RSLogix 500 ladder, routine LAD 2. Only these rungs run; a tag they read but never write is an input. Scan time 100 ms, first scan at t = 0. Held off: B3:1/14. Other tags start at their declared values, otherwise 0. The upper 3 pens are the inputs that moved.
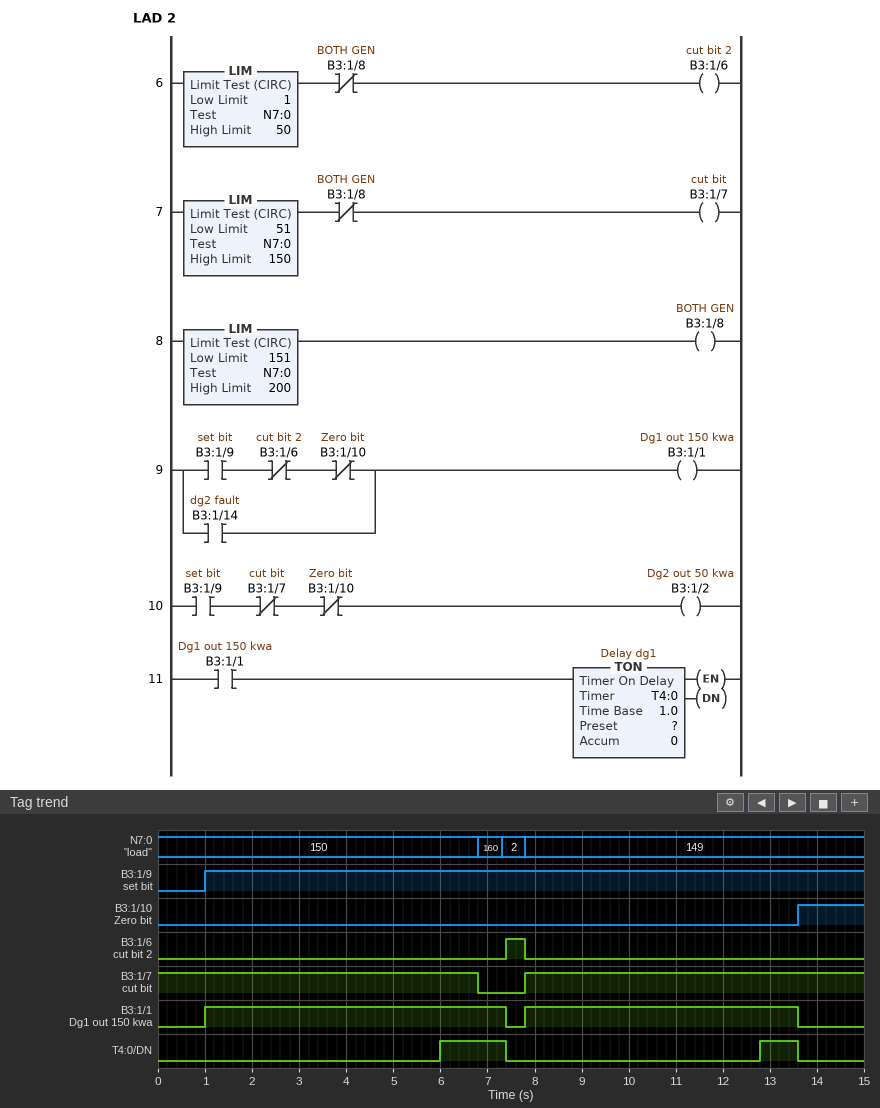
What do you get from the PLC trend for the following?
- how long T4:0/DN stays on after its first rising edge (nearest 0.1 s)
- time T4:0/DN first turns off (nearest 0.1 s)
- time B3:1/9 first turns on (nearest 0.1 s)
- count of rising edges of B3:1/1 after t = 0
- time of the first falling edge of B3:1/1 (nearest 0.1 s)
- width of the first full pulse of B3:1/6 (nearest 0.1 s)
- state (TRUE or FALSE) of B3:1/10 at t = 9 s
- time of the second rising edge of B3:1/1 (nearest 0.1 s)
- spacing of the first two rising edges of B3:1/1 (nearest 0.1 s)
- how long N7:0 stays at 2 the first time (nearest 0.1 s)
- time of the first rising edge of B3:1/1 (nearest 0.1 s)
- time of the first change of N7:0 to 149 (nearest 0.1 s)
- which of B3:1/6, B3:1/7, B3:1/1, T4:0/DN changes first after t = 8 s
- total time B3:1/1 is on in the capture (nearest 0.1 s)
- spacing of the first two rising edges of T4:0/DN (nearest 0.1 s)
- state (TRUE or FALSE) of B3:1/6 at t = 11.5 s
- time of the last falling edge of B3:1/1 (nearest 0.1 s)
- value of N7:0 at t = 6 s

1.4 s
7.4 s
1.0 s
2
7.4 s
0.4 s
FALSE
7.8 s
6.8 s
0.5 s
1.0 s
7.8 s
T4:0/DN
12.2 s
6.8 s
FALSE
13.6 s
150
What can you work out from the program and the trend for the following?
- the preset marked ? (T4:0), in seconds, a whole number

5 s
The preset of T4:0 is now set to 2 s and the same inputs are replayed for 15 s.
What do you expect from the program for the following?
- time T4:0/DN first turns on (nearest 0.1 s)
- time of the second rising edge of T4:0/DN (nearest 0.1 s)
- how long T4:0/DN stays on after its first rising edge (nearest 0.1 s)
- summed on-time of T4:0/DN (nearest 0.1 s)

3.0 s
9.8 s
4.4 s
8.2 s
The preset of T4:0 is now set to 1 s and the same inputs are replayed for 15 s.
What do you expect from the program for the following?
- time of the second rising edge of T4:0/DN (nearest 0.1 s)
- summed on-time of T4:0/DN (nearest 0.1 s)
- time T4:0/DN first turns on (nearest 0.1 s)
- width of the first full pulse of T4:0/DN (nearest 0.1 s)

8.8 s
10.2 s
2.0 s
5.4 s
